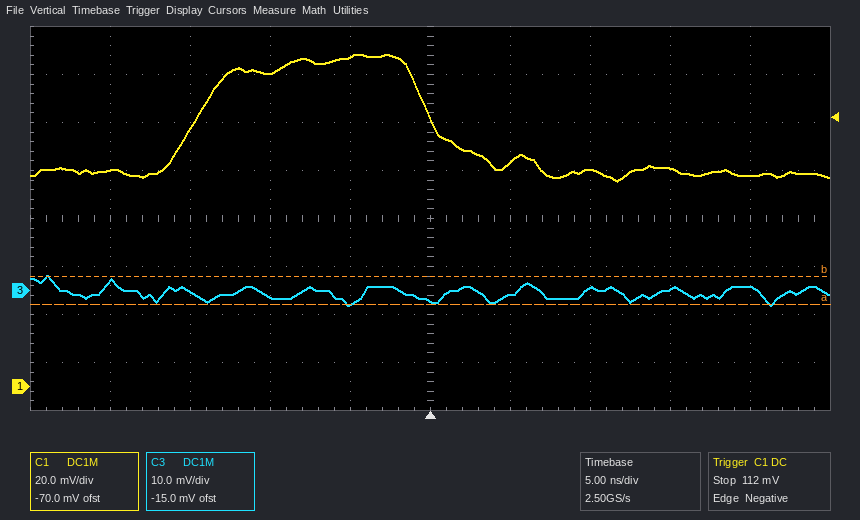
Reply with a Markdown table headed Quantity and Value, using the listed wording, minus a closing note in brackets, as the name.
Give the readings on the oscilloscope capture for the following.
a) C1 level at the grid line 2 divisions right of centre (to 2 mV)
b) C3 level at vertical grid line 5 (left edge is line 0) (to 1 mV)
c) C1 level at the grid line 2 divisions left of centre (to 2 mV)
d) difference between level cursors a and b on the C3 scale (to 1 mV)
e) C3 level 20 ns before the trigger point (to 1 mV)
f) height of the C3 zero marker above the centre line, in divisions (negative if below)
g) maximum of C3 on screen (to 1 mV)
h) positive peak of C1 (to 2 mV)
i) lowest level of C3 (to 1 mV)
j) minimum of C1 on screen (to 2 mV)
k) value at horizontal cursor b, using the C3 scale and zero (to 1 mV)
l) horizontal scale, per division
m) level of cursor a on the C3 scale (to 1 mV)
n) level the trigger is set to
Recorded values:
| Quantity | Value |
|---|---|
| C1 level at the grid line 2 divisions right of centre | 90 mV |
| C3 level at vertical grid line 5 (left edge is line 0) | -2 mV |
| C1 level at the grid line 2 divisions left of centre | 130 mV |
| difference between level cursors a and b on the C3 scale | 6 mV |
| C3 level 20 ns before the trigger point | 2 mV |
| height of the C3 zero marker above the centre line, in divisions | -1.5 div |
| maximum of C3 on screen | 3 mV |
| positive peak of C1 | 138 mV |
| lowest level of C3 | -3 mV |
| minimum of C1 on screen | 86 mV |
| value at horizontal cursor b, using the C3 scale and zero | 3 mV |
| horizontal scale, per division | 5 ns |
| level of cursor a on the C3 scale | -3 mV |
| level the trigger is set to | 112 mV |
